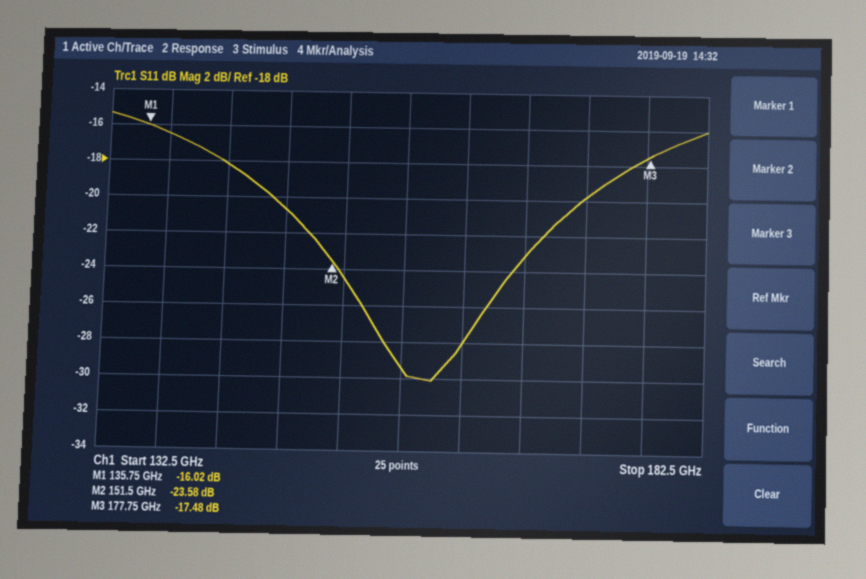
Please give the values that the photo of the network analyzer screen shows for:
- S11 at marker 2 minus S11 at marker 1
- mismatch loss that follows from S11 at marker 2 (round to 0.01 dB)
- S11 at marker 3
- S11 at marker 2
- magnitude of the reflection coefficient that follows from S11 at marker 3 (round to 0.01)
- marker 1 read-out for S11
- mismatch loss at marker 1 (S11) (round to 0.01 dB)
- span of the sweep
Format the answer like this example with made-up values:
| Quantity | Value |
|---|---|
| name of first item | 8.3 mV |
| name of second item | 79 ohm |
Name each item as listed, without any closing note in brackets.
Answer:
| Quantity | Value |
|---|---|
| S11 at marker 2 minus S11 at marker 1 | -7.56 dB |
| mismatch loss that follows from S11 at marker 2 | 0.02 dB |
| S11 at marker 3 | -17.48 dB |
| S11 at marker 2 | -23.58 dB |
| magnitude of the reflection coefficient that follows from S11 at marker 3 | 0.13 |
| marker 1 read-out for S11 | -16.02 dB |
| mismatch loss at marker 1 (S11) | 0.11 dB |
| span of the sweep | 50 GHz |
